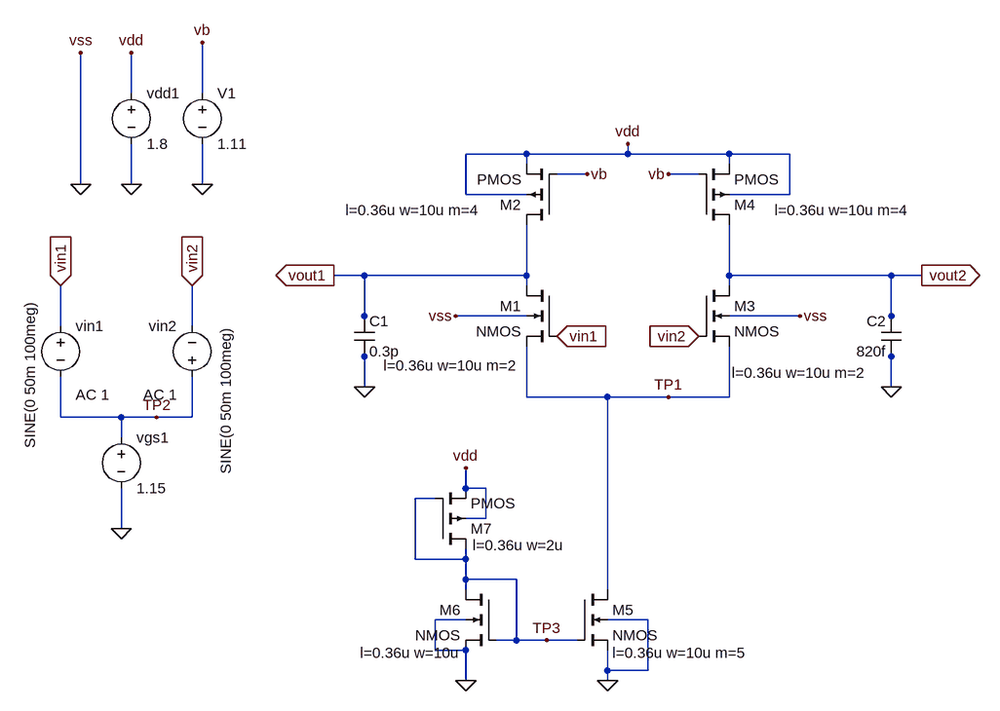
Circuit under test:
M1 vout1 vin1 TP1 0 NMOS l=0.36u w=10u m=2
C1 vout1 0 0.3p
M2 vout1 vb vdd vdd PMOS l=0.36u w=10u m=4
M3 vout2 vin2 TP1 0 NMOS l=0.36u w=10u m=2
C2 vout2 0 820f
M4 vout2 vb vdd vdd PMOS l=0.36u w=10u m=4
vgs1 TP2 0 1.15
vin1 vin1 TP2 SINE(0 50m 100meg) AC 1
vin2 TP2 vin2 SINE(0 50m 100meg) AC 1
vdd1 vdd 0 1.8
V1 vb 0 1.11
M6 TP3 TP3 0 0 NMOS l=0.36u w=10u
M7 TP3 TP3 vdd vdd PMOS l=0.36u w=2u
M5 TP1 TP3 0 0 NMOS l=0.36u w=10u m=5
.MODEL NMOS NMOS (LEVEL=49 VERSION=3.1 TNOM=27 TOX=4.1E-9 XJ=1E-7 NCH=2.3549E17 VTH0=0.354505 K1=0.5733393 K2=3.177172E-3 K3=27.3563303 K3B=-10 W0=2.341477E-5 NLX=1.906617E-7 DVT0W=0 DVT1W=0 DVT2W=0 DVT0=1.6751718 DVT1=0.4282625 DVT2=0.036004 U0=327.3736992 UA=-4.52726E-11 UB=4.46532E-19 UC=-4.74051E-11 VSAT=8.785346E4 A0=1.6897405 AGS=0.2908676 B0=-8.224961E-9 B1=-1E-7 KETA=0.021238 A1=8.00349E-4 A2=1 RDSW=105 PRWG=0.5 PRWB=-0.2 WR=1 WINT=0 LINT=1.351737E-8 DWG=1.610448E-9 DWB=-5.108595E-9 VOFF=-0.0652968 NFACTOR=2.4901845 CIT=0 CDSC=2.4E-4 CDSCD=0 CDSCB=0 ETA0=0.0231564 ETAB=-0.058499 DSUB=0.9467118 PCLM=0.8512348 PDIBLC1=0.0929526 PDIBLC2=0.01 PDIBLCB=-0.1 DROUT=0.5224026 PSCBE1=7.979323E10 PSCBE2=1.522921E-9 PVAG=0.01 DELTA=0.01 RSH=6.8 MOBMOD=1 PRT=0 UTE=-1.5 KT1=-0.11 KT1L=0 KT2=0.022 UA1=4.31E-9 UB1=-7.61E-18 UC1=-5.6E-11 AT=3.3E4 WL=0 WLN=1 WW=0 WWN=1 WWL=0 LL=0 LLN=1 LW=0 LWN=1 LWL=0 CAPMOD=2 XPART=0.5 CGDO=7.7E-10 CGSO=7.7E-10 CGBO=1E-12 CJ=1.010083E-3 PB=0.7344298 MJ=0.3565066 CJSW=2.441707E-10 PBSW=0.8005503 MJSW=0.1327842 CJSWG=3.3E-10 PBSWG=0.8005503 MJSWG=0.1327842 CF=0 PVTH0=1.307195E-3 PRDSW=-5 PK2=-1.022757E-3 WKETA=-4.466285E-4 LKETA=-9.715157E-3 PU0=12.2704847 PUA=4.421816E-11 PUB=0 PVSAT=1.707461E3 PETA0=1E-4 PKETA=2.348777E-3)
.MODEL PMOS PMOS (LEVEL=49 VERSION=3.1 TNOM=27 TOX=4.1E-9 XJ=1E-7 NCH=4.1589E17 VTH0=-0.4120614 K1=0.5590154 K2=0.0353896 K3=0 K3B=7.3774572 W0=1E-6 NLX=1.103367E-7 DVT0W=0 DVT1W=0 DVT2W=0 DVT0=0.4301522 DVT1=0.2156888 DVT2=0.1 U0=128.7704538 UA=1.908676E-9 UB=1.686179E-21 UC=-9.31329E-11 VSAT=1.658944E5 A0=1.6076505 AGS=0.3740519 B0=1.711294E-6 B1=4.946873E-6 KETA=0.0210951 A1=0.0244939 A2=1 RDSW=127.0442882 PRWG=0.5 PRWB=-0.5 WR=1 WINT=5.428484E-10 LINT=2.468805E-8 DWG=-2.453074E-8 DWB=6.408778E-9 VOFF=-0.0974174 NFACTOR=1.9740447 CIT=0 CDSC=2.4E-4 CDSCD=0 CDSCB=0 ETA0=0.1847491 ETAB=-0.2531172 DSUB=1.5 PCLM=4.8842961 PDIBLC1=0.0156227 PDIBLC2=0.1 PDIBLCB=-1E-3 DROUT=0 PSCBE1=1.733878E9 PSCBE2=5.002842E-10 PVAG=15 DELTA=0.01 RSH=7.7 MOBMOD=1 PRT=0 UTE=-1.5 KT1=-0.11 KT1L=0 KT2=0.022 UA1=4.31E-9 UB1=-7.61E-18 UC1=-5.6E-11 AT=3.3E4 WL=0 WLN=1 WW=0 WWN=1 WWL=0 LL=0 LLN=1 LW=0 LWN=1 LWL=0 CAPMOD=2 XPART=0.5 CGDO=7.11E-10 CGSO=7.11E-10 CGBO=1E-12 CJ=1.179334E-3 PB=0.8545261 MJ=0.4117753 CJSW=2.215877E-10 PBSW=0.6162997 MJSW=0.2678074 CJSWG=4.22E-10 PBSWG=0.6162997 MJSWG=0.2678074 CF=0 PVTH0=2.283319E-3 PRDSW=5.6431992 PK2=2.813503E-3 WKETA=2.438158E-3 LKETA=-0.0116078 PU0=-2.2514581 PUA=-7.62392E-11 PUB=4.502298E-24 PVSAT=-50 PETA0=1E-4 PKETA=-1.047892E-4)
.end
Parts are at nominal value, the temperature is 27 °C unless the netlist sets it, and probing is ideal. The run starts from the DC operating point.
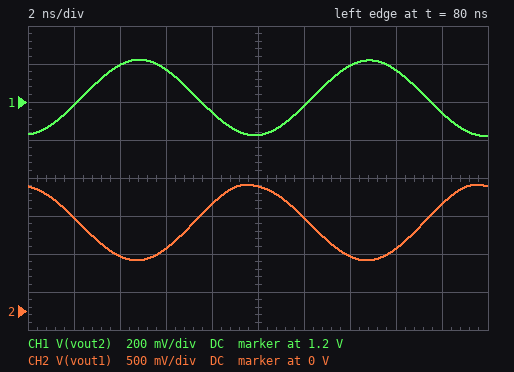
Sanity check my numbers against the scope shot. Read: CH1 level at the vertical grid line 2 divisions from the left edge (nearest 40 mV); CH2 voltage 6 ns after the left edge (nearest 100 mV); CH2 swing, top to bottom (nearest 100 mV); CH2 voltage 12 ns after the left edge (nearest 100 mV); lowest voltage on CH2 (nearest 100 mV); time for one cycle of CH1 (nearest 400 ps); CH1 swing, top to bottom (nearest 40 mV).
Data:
1.40 V
800 mV
1.0 V
1.2 V
700 mV
10.0 ns
400 mV
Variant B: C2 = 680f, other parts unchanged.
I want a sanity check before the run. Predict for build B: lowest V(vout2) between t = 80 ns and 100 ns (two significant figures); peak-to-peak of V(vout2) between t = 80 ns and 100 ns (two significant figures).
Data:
980 mV
470 mV
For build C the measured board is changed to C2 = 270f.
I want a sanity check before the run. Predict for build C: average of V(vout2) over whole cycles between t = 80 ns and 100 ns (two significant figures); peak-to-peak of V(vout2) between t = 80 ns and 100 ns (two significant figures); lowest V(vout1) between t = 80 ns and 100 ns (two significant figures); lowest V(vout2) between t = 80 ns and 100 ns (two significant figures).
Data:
1.1 V
1.0 V
650 mV
620 mV
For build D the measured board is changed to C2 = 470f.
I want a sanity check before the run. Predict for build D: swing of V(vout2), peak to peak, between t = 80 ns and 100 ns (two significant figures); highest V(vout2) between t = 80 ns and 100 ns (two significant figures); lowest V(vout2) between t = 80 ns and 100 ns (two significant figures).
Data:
660 mV
1.5 V
880 mV
